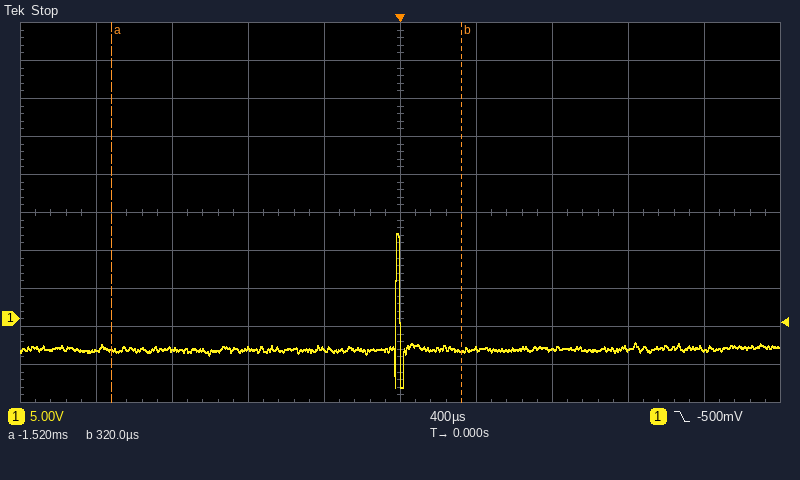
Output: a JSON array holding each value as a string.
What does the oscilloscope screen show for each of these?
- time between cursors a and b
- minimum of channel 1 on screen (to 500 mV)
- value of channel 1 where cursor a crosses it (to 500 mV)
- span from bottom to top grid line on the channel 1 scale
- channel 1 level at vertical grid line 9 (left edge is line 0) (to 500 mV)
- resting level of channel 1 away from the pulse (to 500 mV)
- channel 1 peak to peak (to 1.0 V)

["1.84 ms", "-9.0 V", "-4.0 V", "50 V", "-4.0 V", "-4.0 V", "20.0 V"]
